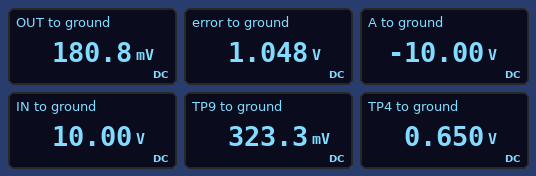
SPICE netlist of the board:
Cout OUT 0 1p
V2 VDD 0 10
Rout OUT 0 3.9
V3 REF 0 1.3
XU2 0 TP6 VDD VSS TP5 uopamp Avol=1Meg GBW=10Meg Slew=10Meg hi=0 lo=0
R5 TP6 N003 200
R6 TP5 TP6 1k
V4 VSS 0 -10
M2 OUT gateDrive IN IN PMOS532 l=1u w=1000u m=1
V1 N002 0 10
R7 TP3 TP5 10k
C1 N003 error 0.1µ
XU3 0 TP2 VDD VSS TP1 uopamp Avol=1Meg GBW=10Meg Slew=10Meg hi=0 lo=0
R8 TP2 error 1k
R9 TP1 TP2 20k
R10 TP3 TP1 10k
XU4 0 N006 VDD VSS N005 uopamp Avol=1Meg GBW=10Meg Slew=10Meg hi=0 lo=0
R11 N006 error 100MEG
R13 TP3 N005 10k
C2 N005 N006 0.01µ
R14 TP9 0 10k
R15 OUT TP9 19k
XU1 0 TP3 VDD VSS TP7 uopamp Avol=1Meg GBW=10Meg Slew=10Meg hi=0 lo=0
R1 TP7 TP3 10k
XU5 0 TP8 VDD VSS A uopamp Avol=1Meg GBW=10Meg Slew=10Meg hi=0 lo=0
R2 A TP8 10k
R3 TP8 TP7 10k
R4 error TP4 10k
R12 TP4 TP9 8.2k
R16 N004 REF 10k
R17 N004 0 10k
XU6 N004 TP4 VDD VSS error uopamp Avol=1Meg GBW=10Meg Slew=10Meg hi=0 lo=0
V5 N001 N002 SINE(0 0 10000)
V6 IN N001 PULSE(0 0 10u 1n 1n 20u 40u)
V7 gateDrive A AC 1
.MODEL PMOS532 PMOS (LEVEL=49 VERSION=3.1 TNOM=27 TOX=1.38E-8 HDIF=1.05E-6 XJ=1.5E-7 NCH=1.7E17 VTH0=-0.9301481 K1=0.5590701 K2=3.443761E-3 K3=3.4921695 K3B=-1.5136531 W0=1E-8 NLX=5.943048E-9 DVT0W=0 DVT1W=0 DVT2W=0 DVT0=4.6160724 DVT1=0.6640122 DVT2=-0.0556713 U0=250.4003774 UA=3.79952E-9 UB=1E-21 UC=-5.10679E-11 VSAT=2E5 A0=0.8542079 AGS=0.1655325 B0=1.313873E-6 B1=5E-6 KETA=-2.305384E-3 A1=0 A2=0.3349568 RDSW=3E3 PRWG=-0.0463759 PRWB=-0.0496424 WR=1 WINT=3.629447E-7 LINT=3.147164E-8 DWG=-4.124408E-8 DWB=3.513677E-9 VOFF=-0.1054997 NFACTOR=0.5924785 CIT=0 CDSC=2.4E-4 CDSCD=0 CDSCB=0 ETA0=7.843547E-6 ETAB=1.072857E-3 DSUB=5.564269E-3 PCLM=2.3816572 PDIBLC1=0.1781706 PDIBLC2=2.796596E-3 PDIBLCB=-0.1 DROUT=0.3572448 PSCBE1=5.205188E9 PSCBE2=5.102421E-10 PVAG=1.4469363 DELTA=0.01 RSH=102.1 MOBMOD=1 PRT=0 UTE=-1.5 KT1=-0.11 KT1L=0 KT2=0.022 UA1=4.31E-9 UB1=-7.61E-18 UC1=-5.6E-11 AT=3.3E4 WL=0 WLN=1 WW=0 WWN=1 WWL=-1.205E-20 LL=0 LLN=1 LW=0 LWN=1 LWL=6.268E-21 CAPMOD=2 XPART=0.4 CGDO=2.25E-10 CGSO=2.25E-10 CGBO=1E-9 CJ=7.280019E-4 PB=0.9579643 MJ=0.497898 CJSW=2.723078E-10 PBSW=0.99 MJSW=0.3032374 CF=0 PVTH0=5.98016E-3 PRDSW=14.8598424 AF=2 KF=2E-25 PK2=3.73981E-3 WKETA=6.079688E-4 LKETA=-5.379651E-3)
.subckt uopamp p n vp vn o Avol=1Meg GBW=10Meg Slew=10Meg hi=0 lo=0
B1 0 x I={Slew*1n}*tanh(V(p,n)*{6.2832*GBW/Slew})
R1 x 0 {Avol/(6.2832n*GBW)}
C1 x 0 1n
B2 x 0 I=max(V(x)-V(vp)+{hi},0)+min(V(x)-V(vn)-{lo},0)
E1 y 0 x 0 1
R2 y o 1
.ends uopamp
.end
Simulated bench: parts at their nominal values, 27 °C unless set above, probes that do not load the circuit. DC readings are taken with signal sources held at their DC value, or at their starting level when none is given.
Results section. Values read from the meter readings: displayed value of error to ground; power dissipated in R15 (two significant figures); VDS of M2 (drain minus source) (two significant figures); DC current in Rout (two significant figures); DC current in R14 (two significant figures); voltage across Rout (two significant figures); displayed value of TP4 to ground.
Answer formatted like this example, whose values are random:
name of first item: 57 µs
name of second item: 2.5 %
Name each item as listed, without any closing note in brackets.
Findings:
displayed value of error to ground: 1.048 V
power dissipated in R15: 1.1 µW
VDS of M2 (drain minus source): -9.8 V
DC current in Rout: 46 mA
DC current in R14: 32 µA
voltage across Rout: 180 mV
displayed value of TP4 to ground: 0.650 V
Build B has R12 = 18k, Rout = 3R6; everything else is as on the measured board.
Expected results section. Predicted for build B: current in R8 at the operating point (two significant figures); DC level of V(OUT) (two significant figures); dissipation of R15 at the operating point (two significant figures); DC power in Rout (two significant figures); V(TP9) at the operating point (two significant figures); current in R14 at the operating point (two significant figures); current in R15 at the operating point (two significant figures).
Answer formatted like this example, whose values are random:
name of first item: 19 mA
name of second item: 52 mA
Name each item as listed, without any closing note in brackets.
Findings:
current in R8 at the operating point: 520 µA
DC level of V(OUT): 170 mV
dissipation of R15 at the operating point: 120 nW
DC power in Rout: 7.8 mW
V(TP9) at the operating point: 220 mV
current in R14 at the operating point: 22 µA
current in R15 at the operating point: 2.6 µA
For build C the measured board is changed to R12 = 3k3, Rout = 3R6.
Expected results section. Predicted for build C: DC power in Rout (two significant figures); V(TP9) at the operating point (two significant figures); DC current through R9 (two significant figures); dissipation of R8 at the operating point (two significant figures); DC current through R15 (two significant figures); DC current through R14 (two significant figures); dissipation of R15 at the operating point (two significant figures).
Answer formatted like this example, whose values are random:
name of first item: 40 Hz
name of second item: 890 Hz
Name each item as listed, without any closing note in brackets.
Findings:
DC power in Rout: 7.8 mW
V(TP9) at the operating point: 450 mV
DC current through R9: 540 µA
dissipation of R8 at the operating point: 290 µW
DC current through R15: 15 µA
DC current through R14: 45 µA
dissipation of R15 at the operating point: 4.3 µW
